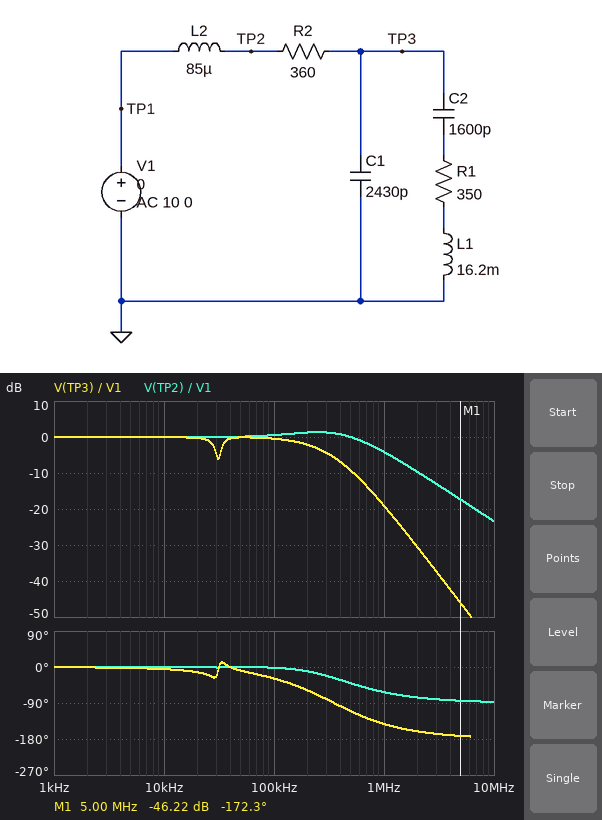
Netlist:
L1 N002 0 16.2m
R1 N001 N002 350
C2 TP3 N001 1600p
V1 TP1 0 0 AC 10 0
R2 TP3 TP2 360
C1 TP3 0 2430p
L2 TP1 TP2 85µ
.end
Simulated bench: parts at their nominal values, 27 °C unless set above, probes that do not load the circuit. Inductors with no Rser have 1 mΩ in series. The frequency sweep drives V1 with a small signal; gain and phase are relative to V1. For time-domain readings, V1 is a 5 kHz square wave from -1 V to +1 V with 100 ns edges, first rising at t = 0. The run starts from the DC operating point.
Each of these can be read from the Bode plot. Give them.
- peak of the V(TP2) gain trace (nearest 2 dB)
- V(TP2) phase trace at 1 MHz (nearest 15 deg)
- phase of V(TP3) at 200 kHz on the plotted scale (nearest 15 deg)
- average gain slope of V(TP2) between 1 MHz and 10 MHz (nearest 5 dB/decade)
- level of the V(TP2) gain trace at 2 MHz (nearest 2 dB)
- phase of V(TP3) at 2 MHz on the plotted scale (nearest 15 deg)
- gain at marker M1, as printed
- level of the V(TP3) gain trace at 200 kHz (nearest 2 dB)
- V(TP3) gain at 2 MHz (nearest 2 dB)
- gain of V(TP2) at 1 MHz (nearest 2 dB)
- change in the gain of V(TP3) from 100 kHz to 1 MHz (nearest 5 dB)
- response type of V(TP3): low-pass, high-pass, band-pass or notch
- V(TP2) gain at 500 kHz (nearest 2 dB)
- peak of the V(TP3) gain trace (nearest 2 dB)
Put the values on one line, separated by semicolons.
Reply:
2 dB; -60 deg; -60 deg; -20 dB/decade; -10 dB; -165 deg; -46.22 dB; -2 dB; -30 dB; -4 dB; -20 dB; low-pass; 0 dB; 0 dB
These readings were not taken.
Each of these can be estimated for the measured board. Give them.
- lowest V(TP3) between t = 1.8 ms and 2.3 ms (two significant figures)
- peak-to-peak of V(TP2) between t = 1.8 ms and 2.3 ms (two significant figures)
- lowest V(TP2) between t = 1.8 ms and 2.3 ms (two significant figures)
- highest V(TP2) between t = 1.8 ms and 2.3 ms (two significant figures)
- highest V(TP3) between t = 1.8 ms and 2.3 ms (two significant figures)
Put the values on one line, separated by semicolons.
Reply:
-1.1 V; 2.6 V; -1.3 V; 1.3 V; 1.1 V
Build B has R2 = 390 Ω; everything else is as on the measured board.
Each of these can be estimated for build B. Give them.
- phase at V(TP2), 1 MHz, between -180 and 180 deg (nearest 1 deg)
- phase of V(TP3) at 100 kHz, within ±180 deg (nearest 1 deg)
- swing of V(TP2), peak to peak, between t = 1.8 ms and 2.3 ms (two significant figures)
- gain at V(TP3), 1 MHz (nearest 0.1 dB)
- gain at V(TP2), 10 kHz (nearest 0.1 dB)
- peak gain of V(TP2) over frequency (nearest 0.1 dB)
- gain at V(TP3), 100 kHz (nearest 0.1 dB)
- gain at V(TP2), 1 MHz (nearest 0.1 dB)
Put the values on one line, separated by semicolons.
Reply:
-60 deg; -31 deg; 2.5 V; -19.4 dB; 0 dB; 1.2 dB; -0.7 dB; -3.8 dB
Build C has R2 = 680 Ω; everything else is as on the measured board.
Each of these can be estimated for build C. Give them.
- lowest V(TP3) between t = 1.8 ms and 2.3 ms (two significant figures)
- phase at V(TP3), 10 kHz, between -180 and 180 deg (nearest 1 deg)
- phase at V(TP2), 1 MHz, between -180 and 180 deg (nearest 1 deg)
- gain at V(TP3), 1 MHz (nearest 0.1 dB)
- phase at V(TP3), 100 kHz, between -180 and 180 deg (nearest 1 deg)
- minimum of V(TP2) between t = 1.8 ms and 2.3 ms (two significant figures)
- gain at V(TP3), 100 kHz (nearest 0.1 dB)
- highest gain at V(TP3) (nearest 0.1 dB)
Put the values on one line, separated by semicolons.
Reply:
-1.2 V; -10 deg; -40 deg; -22.0 dB; -46 deg; -1.1 V; -2.5 dB; 0 dB
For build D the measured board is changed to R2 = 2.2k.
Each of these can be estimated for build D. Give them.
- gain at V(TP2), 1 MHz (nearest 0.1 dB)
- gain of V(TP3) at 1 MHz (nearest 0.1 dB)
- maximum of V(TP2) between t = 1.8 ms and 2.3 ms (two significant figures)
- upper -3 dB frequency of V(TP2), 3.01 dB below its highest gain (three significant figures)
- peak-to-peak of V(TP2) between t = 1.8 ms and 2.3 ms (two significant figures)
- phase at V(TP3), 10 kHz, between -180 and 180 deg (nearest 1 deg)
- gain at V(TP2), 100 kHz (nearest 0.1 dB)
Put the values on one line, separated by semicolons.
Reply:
-0.2 dB; -30.7 dB; 1.0 V; 4.09 MHz; 2.0 V; -30 deg; 0.1 dB
